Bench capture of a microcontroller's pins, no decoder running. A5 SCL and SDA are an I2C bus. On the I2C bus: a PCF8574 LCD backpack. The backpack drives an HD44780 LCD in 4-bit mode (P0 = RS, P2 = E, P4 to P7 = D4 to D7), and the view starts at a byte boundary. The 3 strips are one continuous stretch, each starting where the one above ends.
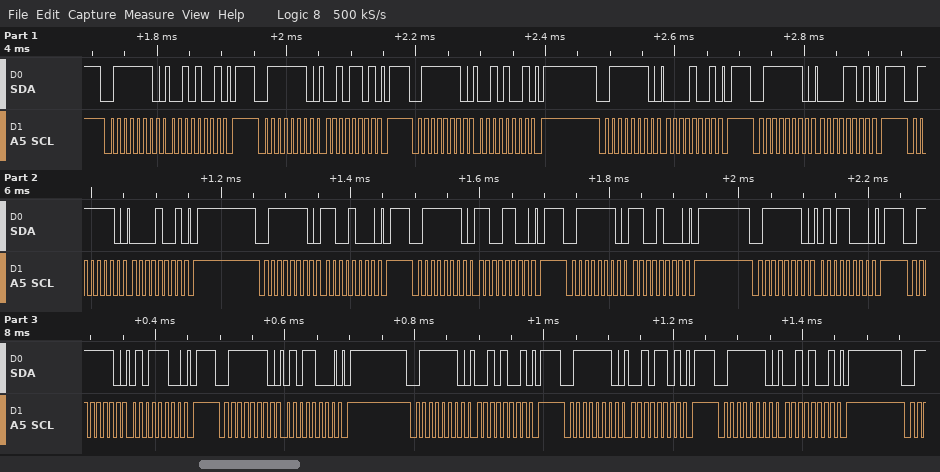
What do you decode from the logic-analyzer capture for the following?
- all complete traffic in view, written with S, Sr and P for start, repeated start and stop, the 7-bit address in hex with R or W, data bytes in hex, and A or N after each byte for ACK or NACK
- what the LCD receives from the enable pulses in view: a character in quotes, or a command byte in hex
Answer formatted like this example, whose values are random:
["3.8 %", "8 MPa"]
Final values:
["S 3FW A 29 A P S 3FW A 2D A P S 3FW A 29 A P S 3FW A 09 A P S 3FW A 0D A P S 3FW A 09 A P S 3FW A C8 A P S 3FW A CC A P S 3FW A C8 A P S 3FW A 58 A P S 3FW A 5C A P S 3FW A 58 A P S 3FW A 29 A P S 3FW A 2D A P S 3FW A 29 A P", "' ' 0xC5"]
